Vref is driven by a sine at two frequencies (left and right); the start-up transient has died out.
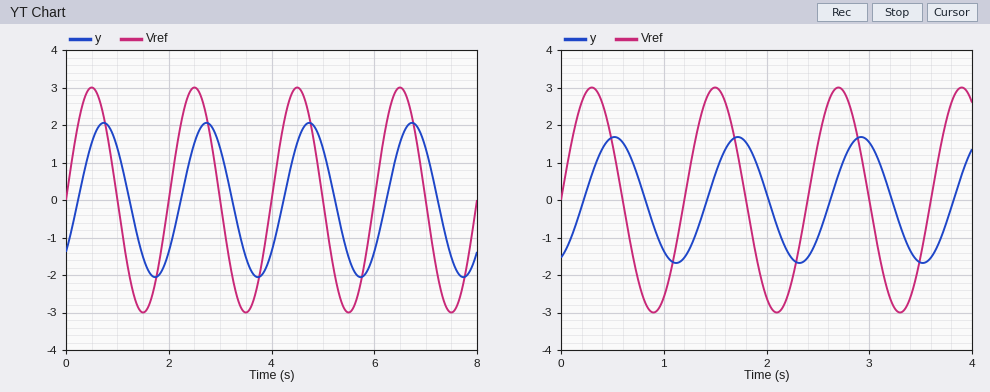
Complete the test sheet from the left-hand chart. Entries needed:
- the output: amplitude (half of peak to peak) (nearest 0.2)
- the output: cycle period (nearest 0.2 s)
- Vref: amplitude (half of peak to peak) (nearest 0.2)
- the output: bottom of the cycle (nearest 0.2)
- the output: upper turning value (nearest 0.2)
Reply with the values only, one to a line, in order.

2.0
2.0 s
3.0
-2.0
2.0
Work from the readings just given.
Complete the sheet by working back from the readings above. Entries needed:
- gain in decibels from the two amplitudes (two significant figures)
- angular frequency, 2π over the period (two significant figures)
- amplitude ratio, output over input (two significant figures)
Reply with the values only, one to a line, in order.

-3.5 dB
3.1 rad/s
0.67
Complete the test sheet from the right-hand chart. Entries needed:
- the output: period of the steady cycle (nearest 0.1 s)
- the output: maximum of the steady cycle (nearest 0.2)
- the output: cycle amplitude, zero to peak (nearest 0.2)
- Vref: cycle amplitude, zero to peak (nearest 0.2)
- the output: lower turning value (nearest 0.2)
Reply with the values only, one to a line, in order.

1.2 s
1.6
1.6
3.0
-1.6
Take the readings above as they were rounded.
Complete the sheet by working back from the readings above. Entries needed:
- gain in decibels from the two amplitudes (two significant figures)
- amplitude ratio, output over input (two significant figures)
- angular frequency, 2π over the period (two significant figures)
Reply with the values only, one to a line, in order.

-5.5 dB
0.53
5.2 rad/s
